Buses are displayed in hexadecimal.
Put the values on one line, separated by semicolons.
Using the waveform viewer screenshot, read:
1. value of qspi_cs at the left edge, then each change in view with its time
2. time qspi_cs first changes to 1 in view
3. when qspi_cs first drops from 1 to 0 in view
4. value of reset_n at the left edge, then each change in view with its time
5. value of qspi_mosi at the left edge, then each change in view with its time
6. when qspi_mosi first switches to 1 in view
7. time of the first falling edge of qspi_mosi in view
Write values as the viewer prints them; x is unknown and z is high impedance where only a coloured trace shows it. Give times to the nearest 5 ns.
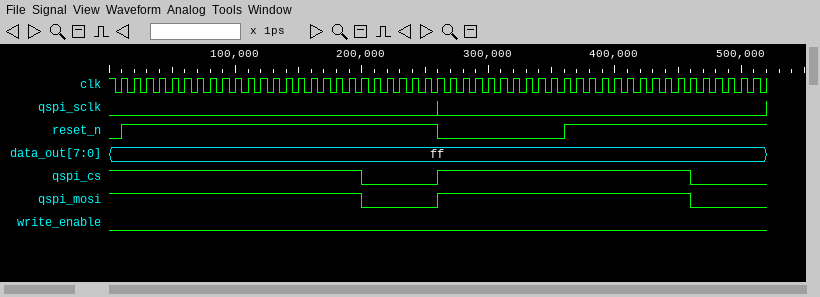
1, 0 at 200 ns, 1 at 260 ns, 0 at 460 ns; 260 ns; 200 ns; 0, 1 at 10 ns, 0 at 260 ns, 1 at 360 ns; 1, 0 at 200 ns, 1 at 260 ns, 0 at 460 ns; 260 ns; 200 ns
